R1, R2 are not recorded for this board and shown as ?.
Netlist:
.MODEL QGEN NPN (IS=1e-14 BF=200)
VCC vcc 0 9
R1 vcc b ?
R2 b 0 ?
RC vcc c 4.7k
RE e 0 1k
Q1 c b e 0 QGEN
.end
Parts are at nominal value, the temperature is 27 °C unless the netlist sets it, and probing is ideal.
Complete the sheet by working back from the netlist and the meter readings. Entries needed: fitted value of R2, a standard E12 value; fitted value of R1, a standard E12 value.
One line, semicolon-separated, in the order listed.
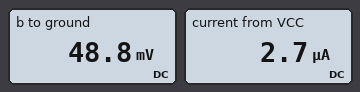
18 kΩ; 3.3 MΩ
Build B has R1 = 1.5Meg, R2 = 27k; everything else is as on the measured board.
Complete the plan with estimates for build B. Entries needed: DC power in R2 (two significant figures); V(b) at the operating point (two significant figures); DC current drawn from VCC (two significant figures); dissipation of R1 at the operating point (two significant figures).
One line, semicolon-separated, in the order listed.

940 nW; 160 mV; 5.9 µA; 52 µW
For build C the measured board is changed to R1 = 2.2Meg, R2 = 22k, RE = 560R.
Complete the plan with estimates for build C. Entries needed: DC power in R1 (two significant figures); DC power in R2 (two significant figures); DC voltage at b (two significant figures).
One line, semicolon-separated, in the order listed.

36 µW; 360 nW; 89 mV
